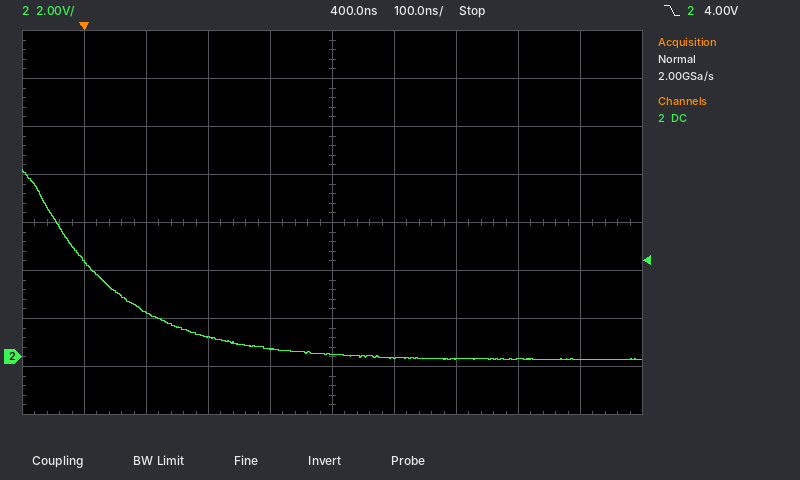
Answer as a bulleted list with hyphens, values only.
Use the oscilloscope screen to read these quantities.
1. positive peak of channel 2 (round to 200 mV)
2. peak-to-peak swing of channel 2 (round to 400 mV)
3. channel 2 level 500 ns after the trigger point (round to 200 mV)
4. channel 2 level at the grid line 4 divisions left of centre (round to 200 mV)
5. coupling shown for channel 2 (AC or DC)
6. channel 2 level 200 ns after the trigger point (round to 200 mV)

- 7.8 V
- 8.0 V
- 0.0 V
- 4.0 V
- DC
- 800 mV
